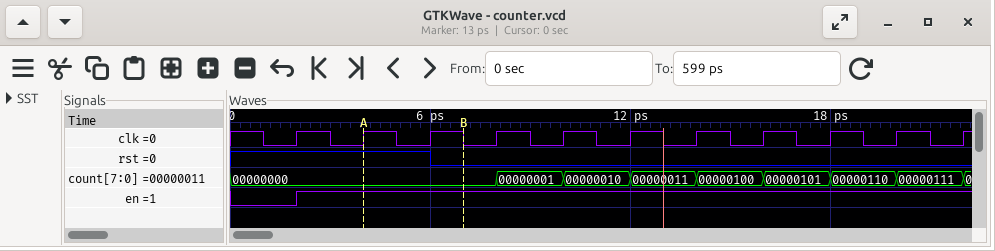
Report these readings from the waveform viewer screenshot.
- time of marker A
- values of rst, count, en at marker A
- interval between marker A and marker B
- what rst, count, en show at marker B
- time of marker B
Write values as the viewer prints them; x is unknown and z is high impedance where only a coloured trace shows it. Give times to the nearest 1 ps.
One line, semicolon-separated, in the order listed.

4 ps; rst=1, count=00000000, en=1; 3 ps; rst=0, count=00000000, en=1; 7 ps
